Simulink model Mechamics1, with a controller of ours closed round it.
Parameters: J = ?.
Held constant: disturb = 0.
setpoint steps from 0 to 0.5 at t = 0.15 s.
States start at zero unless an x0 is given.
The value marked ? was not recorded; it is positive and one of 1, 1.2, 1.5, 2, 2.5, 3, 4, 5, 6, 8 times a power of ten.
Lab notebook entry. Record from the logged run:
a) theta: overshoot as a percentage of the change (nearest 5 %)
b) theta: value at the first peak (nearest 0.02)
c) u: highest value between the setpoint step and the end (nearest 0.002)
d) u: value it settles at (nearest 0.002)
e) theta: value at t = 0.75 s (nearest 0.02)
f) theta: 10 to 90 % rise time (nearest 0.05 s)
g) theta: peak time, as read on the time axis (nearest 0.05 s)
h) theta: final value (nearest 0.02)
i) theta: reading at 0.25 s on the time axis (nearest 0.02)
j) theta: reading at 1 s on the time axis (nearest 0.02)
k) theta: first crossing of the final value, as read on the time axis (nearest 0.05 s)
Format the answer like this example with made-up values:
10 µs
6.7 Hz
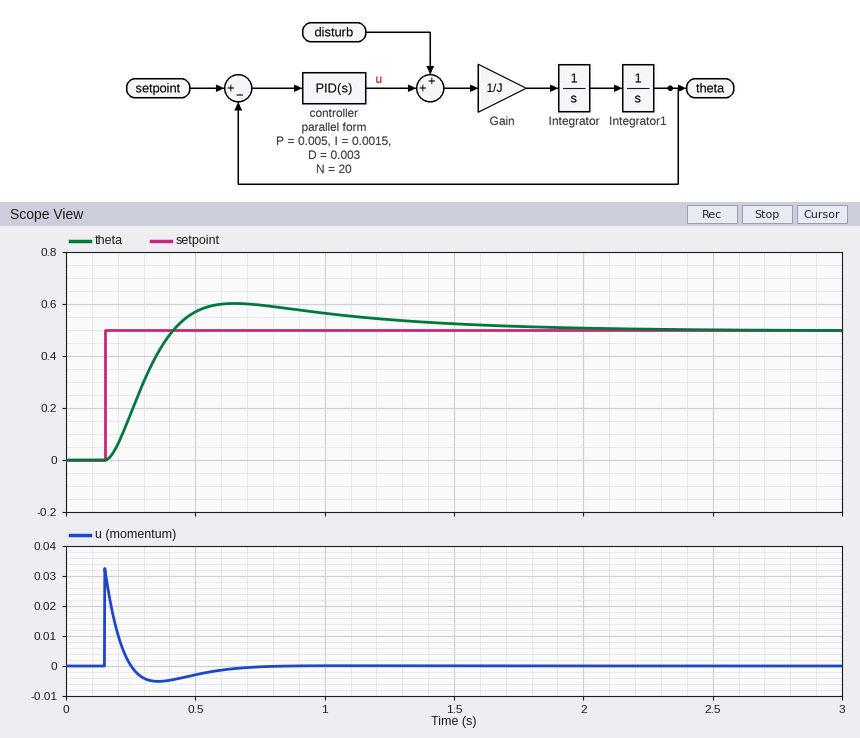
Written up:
20 %
0.60
0.032
0.000
0.60
0.20 s
0.65 s
0.50
0.18
0.56
0.40 s
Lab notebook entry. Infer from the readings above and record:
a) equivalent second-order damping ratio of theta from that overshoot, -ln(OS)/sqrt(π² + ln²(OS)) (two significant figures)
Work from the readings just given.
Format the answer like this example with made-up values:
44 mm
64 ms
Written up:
0.46
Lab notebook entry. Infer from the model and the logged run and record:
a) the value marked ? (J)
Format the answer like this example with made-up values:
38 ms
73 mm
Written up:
0.0005
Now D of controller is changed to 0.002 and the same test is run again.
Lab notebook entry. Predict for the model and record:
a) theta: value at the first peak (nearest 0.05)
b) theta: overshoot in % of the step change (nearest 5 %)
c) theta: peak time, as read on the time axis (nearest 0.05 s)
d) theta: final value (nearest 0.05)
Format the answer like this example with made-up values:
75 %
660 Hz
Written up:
0.65
30 %
0.80 s
0.50
